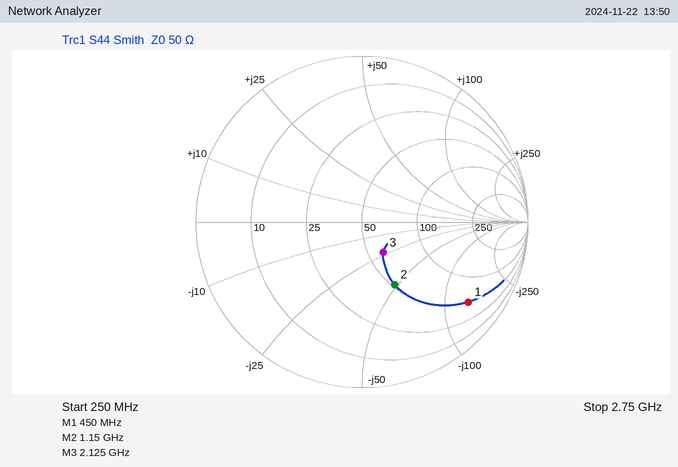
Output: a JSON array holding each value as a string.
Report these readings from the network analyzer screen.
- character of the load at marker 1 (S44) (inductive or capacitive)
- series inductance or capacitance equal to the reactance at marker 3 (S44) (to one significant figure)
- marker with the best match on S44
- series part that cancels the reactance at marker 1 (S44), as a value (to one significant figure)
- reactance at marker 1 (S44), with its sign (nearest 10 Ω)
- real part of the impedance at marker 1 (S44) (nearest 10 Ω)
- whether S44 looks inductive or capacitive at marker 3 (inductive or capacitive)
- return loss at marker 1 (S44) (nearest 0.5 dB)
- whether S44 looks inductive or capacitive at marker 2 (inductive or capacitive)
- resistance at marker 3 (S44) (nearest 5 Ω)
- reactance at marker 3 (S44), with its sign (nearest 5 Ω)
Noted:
["capacitive", "3 pF", "marker 3", "50 nH", "-130 Ω", "50 Ω", "capacitive", "2.0 dB", "capacitive", "60 Ω", "-25 Ω"]
